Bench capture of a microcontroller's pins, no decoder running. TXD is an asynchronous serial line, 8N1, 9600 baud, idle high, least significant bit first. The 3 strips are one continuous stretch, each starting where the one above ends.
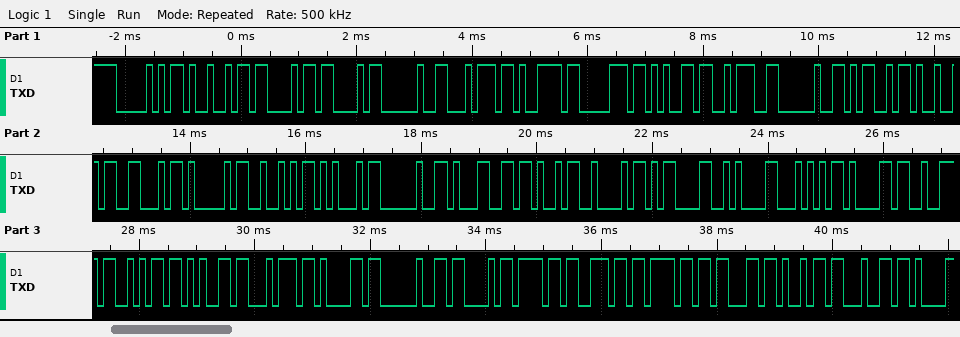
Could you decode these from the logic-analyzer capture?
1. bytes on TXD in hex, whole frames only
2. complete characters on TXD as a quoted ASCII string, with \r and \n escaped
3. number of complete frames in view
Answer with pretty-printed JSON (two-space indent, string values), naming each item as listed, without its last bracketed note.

{
  "bytes on TXD in hex, whole frames only": "0x50 0x49 0x43 0x43 0x20 0x74 0x79 0x70 0x65 0x3A 0x20 0x4D 0x49 0x46 0x41 0x52 0x45 0x20 0x31 0x4B 0x42 0x0D 0x0A 0x54 0x61 0x72 0x6A 0x65 0x74 0x61 0x20 0x43 0x6F 0x6E 0x6F 0x63 0x69 0x64",
  "complete characters on TXD as a quoted ASCII string, with \\r and \\n escaped": "\"PICC type: MIFARE 1KB\\r\\nTarjeta Conocid\"",
  "number of complete frames in view": "38"
}
